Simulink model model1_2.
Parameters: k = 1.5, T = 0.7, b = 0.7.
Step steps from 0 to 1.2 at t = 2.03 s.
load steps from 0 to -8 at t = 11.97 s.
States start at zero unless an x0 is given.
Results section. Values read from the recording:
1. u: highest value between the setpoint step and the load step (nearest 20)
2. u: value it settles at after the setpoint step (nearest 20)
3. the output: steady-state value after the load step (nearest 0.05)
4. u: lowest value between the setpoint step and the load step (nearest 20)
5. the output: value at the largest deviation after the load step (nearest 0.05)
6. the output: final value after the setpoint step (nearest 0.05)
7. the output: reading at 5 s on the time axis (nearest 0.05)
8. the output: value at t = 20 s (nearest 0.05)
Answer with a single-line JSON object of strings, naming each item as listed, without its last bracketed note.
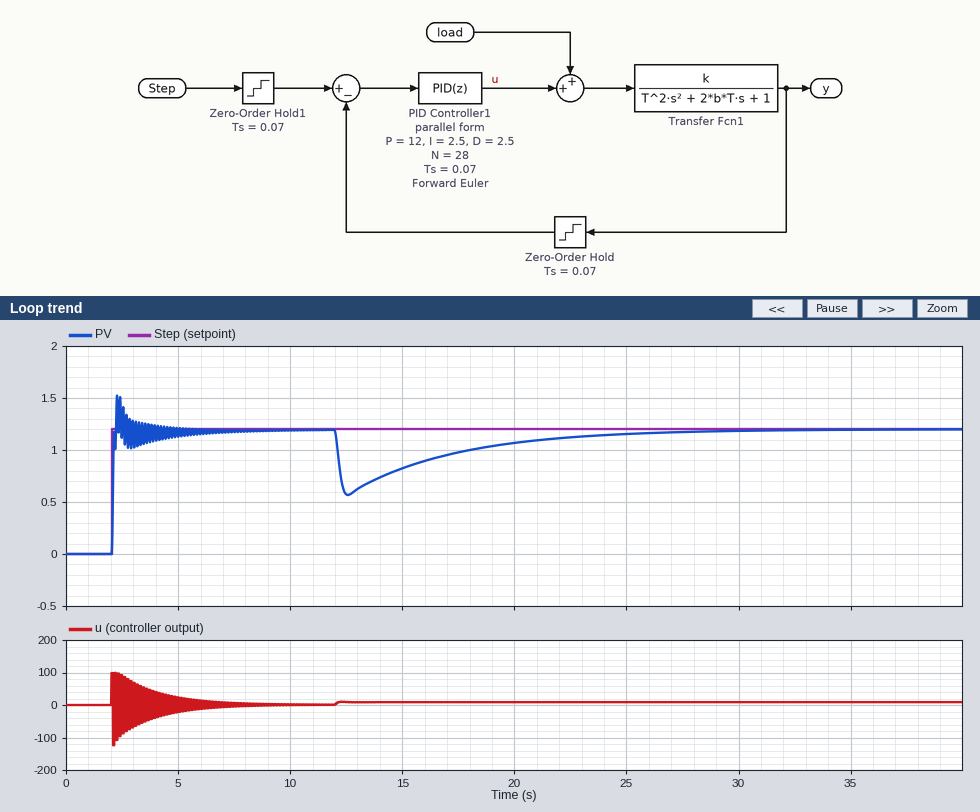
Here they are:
{"u: highest value between the setpoint step and the load step": "100", "u: value it settles at after the setpoint step": "0", "the output: steady-state value after the load step": "1.20", "u: lowest value between the setpoint step and the load step": "-120", "the output: value at the largest deviation after the load step": "0.55", "the output: final value after the setpoint step": "1.20", "the output: reading at 5 s on the time axis": "1.15", "the output: value at t = 20 s": "1.05"}
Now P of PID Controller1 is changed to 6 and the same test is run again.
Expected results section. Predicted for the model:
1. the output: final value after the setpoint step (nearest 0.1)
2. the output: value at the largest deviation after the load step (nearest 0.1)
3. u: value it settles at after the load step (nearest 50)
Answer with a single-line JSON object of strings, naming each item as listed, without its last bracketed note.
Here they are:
{"the output: final value after the setpoint step": "1.2", "the output: value at the largest deviation after the load step": "0.2", "u: value it settles at after the load step": "0"}
